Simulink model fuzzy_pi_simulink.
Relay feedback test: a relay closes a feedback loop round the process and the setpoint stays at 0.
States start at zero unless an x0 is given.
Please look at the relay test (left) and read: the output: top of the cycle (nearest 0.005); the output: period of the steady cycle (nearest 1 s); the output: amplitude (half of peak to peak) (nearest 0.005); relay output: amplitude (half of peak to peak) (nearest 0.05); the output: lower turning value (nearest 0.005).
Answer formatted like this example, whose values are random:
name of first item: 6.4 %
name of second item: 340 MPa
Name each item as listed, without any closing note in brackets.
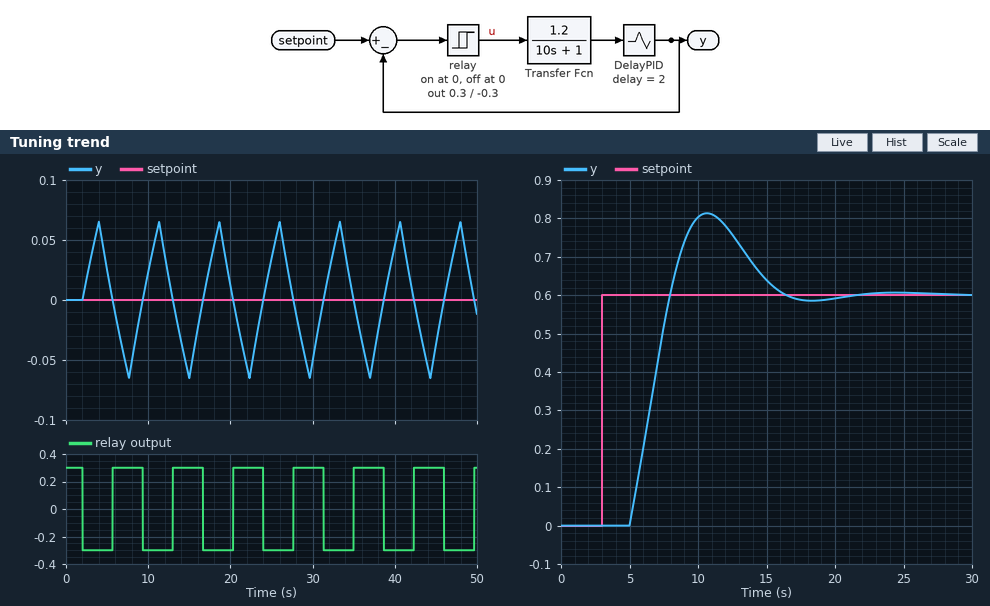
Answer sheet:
the output: top of the cycle: 0.065
the output: period of the steady cycle: 7 s
the output: amplitude (half of peak to peak): 0.065
relay output: amplitude (half of peak to peak): 0.30
the output: lower turning value: -0.065
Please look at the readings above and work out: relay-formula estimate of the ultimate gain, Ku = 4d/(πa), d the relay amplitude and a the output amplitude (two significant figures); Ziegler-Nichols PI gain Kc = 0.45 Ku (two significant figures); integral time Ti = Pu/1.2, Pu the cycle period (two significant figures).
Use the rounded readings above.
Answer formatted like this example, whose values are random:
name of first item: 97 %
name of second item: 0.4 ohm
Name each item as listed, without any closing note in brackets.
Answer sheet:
relay-formula estimate of the ultimate gain, Ku = 4d/(πa), d the relay amplitude and a the output amplitude: 5.9
Ziegler-Nichols PI gain Kc = 0.45 Ku: 2.7
integral time Ti = Pu/1.2, Pu the cycle period: 5.8 s
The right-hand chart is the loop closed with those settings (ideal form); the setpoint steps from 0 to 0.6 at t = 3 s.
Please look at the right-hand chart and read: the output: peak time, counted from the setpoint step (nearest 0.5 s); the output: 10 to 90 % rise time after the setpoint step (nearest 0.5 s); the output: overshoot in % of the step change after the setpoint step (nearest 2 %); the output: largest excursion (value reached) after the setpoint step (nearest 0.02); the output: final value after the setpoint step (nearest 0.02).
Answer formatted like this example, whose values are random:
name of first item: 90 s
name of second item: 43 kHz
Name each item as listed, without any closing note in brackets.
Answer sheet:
the output: peak time, counted from the setpoint step: 7.5 s
the output: 10 to 90 % rise time after the setpoint step: 2.5 s
the output: overshoot in % of the step change after the setpoint step: 36 %
the output: largest excursion (value reached) after the setpoint step: 0.82
the output: final value after the setpoint step: 0.60
